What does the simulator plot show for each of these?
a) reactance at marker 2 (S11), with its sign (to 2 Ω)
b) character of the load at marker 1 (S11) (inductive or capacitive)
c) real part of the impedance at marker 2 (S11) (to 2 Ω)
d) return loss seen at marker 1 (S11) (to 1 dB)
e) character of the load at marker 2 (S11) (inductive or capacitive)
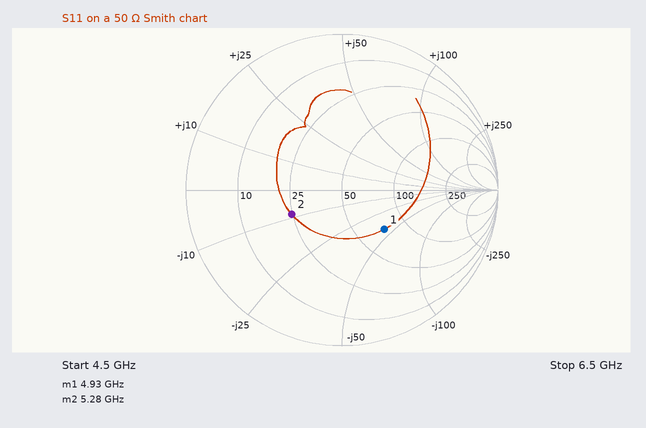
-8 Ω
capacitive
24 Ω
9 dB
capacitive
